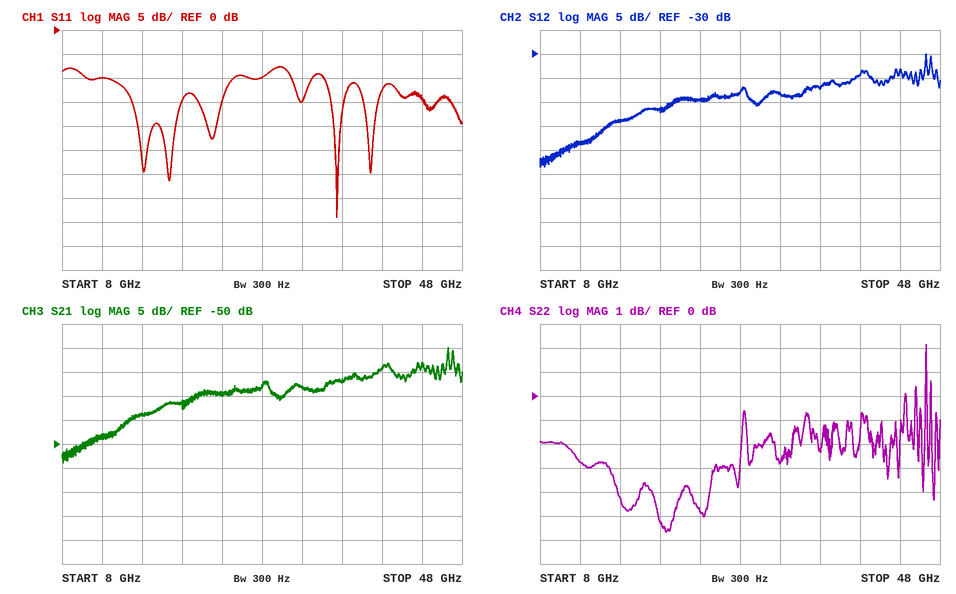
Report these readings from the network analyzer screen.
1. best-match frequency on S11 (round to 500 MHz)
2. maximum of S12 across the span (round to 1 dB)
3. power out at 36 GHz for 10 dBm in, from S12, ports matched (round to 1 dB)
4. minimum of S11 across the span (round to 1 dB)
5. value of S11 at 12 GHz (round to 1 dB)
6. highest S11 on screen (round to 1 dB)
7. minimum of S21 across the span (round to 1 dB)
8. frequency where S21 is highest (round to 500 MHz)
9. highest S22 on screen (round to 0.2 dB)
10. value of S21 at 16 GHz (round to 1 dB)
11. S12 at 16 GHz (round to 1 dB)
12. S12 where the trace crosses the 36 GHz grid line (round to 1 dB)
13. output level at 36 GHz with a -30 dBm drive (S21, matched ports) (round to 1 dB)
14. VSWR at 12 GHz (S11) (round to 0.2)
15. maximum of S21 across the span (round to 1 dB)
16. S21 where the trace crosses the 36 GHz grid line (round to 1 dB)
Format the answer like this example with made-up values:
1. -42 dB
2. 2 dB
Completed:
1. 35.5 GHz
2. -30 dB
3. -27 dBm
4. -39 dB
5. -10 dB
6. -8 dB
7. -54 dB
8. 46.5 GHz
9. 2.2 dB
10. -44 dB
11. -44 dB
12. -37 dB
13. -67 dBm
14. 2.0
15. -30 dB
16. -37 dB
